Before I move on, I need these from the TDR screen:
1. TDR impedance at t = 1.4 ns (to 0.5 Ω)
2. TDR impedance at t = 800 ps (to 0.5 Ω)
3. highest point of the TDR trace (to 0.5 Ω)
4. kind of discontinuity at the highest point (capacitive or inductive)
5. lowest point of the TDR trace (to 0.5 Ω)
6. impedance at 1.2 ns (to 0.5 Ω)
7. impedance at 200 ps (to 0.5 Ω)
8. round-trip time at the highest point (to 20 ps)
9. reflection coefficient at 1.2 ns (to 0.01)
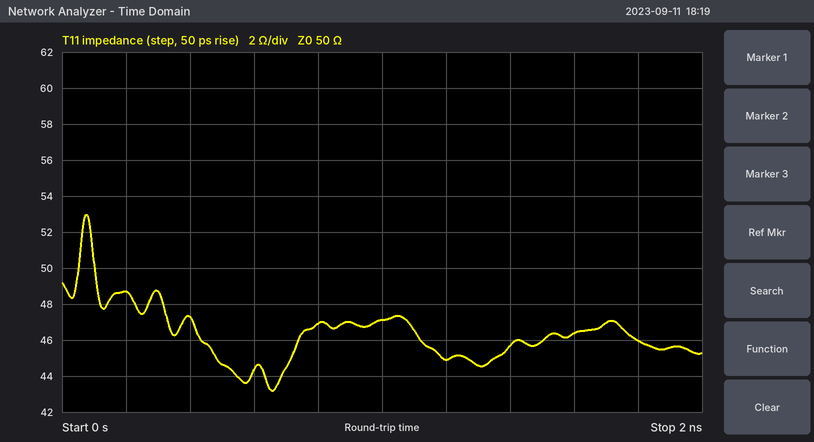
45.5 Ω
47.0 Ω
53.0 Ω
inductive
43.0 Ω
45.0 Ω
48.5 Ω
80 ps
-0.05
